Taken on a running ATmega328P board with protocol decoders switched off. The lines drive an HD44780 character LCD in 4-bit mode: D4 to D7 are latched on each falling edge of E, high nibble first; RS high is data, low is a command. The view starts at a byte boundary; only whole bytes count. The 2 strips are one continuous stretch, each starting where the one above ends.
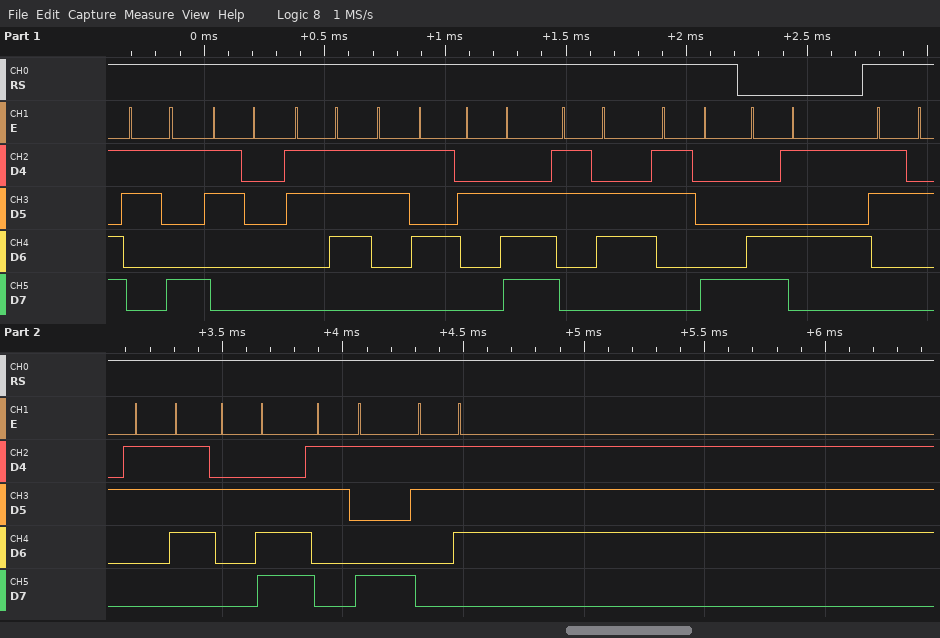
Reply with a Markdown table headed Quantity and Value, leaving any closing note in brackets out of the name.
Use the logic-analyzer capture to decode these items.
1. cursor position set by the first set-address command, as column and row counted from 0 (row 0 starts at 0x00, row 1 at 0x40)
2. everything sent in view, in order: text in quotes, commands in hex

| Quantity | Value |
|---|---|
| cursor position set by the first set-address command, as column and row counted from 0 | column 5, row 1 |
| everything sent in view, in order: text in quotes, commands in hex | "9075.68" 0xC5 "27.97" |
